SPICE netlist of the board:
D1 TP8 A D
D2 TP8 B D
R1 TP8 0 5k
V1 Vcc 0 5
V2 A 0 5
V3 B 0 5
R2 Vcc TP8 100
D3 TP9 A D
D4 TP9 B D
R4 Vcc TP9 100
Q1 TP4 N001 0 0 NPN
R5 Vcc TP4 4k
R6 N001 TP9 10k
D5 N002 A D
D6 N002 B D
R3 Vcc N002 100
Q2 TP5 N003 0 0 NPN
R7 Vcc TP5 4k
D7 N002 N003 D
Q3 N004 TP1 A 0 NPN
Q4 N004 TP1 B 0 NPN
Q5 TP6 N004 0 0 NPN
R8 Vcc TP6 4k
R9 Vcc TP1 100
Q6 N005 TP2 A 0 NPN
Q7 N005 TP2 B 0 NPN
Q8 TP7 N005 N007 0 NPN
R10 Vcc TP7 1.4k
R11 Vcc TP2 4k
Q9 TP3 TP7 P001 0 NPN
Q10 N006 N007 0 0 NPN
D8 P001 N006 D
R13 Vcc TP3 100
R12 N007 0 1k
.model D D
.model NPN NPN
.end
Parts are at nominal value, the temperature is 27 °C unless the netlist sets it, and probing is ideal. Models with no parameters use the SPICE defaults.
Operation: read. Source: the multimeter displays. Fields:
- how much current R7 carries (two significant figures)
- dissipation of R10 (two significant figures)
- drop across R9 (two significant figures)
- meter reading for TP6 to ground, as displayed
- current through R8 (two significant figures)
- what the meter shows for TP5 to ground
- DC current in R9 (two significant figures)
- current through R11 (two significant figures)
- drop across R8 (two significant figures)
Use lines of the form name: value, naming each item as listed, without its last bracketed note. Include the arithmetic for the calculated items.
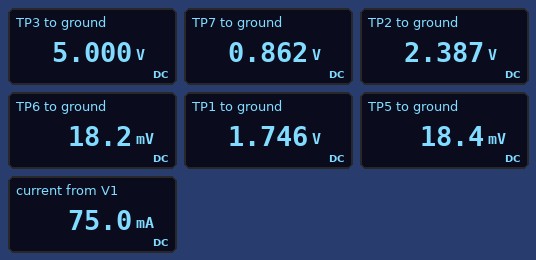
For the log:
how much current R7 carries: (5 V - 18.4 mV) / 4 kΩ = 1.2 mA
dissipation of R10: (5 V - 862 mV)^2 / 1.4 kΩ = 12 mW
drop across R9: 5 V - 1.746 V = 3.3 V
meter reading for TP6 to ground, as displayed: 18.2 mV
current through R8: (5 V - 18.2 mV) / 4 kΩ = 1.2 mA
what the meter shows for TP5 to ground: 18.4 mV
DC current in R9: (5 V - 1.746 V) / 100 Ω = 33 mA
current through R11: (5 V - 2.387 V) / 4 kΩ = 650 µA
drop across R8: 5 V - 18.2 mV = 5.0 V
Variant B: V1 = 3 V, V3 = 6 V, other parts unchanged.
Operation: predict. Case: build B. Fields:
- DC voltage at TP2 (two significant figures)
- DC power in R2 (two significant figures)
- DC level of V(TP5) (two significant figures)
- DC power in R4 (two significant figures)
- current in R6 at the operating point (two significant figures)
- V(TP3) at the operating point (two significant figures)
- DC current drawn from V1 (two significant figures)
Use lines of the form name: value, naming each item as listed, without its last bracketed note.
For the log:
DC voltage at TP2: 2.3 V
DC power in R2: 35 µW
DC level of V(TP5): 19 mV
DC power in R4: 4.8 µW
current in R6 at the operating point: 220 µA
V(TP3) at the operating point: 3.0 V
DC current drawn from V1: 32 mA
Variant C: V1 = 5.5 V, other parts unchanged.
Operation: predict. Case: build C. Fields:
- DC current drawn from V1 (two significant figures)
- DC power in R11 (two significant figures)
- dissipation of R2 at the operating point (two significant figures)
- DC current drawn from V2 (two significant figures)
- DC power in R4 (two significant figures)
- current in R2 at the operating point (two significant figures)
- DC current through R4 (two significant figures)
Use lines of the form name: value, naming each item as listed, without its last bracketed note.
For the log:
DC current drawn from V1: 86 mA
DC power in R11: 2.4 mW
dissipation of R2 at the operating point: 120 µW
DC current drawn from V2: 19 mA
DC power in R4: 22 µW
current in R2 at the operating point: 1.1 mA
DC current through R4: 470 µA
